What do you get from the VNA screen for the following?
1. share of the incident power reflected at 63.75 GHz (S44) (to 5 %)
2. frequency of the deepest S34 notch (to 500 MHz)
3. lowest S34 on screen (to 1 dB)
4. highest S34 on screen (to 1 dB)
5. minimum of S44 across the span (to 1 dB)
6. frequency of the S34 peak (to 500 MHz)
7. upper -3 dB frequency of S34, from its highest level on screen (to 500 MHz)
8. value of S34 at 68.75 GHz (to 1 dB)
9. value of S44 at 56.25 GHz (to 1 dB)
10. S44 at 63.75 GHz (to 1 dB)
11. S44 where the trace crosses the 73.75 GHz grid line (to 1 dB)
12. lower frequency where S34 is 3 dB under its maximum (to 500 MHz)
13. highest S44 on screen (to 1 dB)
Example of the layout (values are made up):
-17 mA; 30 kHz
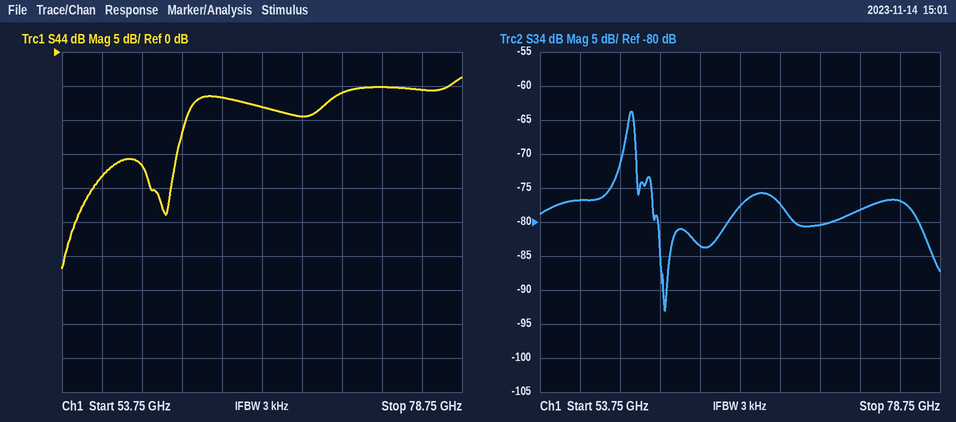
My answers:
20 %; 61.5 GHz; -93 dB; -64 dB; -32 dB; 59.5 GHz; 59.5 GHz; -77 dB; -18 dB; -7 dB; -5 dB; 59.0 GHz; -4 dB
